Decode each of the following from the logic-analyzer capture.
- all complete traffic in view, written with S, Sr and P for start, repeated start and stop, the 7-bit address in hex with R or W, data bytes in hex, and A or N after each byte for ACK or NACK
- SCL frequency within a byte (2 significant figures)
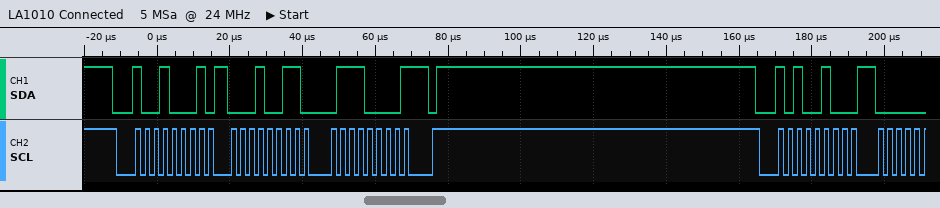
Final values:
S 48R A 13 A 70 N P S 52W A
400 kHz
